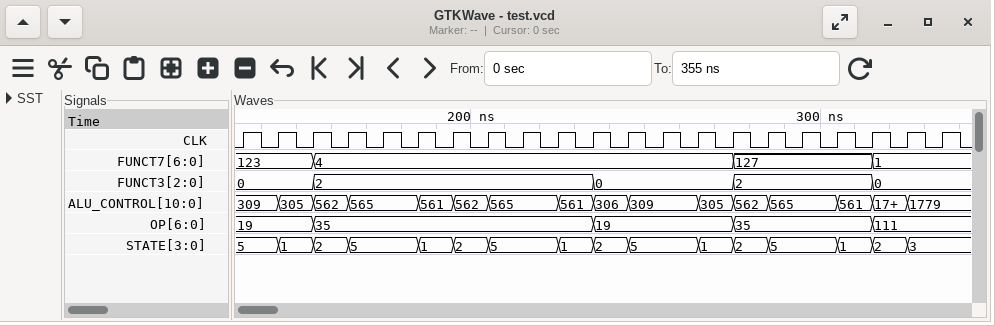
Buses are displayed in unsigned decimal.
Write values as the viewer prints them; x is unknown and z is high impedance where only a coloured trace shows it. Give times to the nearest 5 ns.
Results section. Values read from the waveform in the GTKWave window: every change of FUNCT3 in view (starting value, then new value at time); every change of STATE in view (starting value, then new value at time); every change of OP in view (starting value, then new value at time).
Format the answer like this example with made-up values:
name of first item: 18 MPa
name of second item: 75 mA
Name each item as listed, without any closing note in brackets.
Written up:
every change of FUNCT3 in view: 0, 2 at 155 ns, 0 at 235 ns, 2 at 275 ns, 0 at 315 ns
every change of STATE in view: 5, 1 at 145 ns, 2 at 155 ns, 5 at 165 ns, 1 at 185 ns, 2 at 195 ns, 5 at 205 ns, 1 at 225 ns, 2 at 235 ns, 5 at 245 ns, 1 at 265 ns, 2 at 275 ns, 5 at 285 ns, 1 at 305 ns, 2 at 315 ns, 3 at 325 ns
every change of OP in view: 19, 35 at 155 ns, 19 at 235 ns, 35 at 275 ns, 111 at 315 ns
